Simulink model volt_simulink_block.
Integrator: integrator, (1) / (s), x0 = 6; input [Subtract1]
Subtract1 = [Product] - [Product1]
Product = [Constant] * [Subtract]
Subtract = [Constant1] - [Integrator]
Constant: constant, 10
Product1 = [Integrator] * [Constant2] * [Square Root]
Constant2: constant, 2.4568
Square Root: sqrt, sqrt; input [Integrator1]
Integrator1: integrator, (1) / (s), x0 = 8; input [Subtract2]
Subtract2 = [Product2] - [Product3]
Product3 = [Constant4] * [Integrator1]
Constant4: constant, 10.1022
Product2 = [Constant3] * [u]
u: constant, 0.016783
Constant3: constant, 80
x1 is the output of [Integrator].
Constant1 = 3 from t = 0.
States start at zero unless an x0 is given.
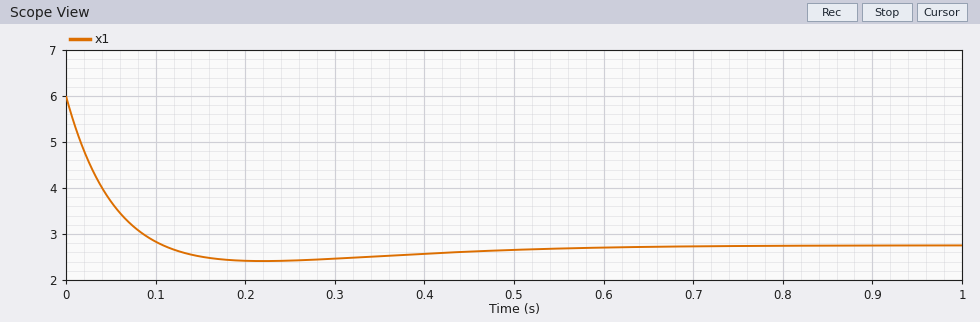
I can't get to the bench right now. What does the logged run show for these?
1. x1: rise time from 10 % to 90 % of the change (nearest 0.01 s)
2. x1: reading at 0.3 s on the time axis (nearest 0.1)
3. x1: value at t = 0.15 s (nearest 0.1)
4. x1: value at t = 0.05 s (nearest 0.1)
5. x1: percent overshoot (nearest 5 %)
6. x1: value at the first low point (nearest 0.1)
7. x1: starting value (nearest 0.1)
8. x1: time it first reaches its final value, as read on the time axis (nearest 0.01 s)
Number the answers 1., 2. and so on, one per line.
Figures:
1. 0.08 s
2. 2.5
3. 2.5
4. 3.7
5. 10 %
6. 2.4
7. 6.0
8. 0.11 s
